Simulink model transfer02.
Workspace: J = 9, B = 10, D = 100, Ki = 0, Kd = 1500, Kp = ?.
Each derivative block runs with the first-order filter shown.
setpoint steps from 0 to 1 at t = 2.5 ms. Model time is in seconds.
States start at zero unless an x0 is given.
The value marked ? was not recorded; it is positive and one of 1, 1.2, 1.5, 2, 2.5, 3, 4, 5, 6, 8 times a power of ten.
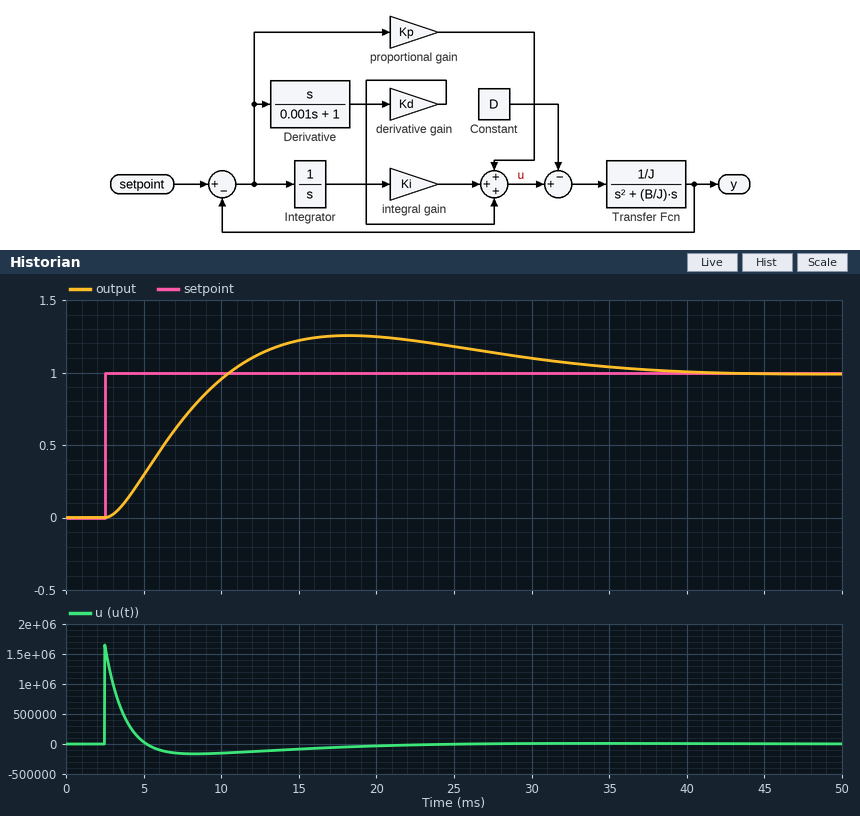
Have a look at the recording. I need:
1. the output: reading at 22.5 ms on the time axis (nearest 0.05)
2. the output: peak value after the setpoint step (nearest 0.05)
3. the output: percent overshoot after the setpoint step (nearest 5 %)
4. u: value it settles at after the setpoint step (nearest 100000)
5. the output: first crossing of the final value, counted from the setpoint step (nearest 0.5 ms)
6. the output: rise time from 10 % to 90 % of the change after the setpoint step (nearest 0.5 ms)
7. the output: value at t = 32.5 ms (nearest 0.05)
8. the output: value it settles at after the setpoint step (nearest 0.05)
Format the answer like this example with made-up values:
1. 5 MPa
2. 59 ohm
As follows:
1. 1.20
2. 1.25
3. 25 %
4. 0
5. 8.0 ms
6. 5.5 ms
7. 1.05
8. 1.00
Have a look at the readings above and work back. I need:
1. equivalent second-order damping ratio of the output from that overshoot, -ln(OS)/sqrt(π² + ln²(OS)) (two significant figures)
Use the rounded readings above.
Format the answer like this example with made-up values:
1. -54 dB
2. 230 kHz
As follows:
1. 0.40
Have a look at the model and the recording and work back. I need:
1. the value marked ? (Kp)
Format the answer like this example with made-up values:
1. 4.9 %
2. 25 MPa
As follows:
1. 150000
